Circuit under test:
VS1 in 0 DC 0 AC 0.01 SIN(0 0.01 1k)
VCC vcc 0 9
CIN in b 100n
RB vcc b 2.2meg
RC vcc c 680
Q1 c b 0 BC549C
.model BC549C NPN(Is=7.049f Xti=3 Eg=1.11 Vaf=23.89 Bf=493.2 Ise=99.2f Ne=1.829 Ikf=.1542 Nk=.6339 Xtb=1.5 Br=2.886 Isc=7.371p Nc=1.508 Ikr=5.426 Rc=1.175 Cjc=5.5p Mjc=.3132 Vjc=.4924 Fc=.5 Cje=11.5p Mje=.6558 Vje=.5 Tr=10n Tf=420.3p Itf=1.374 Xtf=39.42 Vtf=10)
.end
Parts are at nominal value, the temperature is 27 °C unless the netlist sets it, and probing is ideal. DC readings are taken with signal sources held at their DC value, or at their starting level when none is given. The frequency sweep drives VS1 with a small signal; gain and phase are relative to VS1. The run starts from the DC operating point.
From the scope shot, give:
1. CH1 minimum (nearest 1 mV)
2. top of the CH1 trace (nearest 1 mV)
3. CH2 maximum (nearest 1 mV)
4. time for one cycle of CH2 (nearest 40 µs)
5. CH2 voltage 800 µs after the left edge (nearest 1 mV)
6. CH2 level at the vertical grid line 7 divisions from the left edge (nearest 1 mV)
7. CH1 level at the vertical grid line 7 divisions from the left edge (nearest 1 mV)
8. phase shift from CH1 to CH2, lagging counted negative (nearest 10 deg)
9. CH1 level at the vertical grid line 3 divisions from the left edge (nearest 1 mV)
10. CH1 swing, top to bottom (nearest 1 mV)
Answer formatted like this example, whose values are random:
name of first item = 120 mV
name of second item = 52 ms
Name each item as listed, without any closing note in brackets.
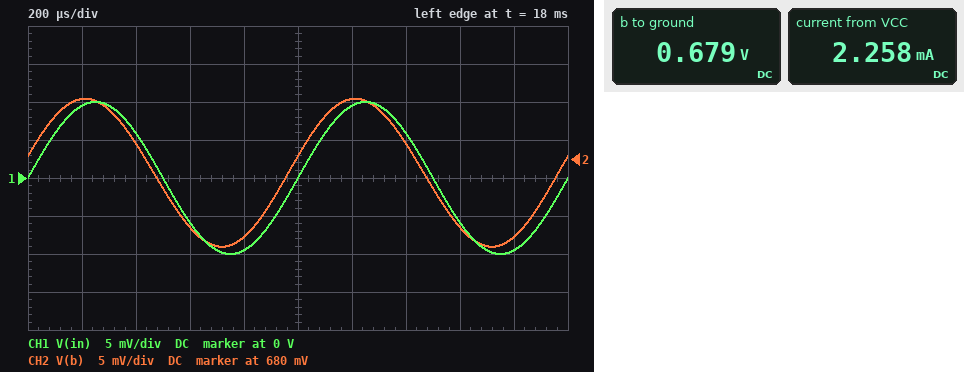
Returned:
CH1 minimum = -10 mV
top of the CH1 trace = 10 mV
CH2 maximum = 688 mV
time for one cycle of CH2 = 1.00 ms
CH2 voltage 800 µs after the left edge = 670 mV
CH2 level at the vertical grid line 7 divisions from the left edge = 682 mV
CH1 level at the vertical grid line 7 divisions from the left edge = 6 mV
phase shift from CH1 to CH2, lagging counted negative = 10 deg
CH1 level at the vertical grid line 3 divisions from the left edge = -6 mV
CH1 swing, top to bottom = 20 mV
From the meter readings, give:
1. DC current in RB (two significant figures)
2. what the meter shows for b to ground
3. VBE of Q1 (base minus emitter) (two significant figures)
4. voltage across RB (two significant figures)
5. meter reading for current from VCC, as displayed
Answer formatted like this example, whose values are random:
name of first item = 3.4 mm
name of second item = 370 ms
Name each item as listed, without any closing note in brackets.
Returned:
DC current in RB = 3.8 µA
what the meter shows for b to ground = 0.679 V
VBE of Q1 (base minus emitter) = 680 mV
voltage across RB = 8.3 V
meter reading for current from VCC, as displayed = 2.258 mA
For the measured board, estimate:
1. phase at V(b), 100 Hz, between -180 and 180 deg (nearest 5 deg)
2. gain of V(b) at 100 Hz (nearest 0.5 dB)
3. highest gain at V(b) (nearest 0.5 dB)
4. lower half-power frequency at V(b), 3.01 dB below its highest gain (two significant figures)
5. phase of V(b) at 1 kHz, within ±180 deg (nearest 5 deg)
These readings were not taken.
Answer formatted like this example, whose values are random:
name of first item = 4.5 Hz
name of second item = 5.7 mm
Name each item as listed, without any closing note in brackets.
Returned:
phase at V(b), 100 Hz, between -180 and 180 deg = 65 deg
gain of V(b) at 100 Hz = -8.0 dB
highest gain at V(b) = 0 dB
lower half-power frequency at V(b), 3.01 dB below its highest gain = 230 Hz
phase of V(b) at 1 kHz, within ±180 deg = 15 deg
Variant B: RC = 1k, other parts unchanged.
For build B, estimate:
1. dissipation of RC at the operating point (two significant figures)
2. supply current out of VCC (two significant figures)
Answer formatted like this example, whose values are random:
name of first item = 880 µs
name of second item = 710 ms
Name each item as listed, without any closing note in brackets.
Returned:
dissipation of RC at the operating point = 4.9 mW
supply current out of VCC = 2.2 mA
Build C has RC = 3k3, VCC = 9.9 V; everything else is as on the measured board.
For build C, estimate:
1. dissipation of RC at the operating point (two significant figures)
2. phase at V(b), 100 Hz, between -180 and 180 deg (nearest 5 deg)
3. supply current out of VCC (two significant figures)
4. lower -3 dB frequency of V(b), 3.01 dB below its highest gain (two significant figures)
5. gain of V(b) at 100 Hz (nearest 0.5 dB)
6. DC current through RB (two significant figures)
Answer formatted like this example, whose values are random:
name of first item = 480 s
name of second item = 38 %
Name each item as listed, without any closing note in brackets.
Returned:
dissipation of RC at the operating point = 15 mW
phase at V(b), 100 Hz, between -180 and 180 deg = 70 deg
supply current out of VCC = 2.1 mA
lower -3 dB frequency of V(b), 3.01 dB below its highest gain = 250 Hz
gain of V(b) at 100 Hz = -8.5 dB
DC current through RB = 4.2 µA
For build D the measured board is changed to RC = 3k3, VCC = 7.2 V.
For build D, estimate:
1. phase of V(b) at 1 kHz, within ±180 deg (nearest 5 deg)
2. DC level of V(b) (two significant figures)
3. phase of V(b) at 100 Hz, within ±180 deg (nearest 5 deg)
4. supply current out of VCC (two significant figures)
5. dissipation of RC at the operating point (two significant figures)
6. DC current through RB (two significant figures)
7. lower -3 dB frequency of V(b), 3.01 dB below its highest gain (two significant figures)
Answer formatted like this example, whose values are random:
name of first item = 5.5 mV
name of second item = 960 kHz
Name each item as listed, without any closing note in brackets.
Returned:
phase of V(b) at 1 kHz, within ±180 deg = 10 deg
DC level of V(b) = 670 mV
phase of V(b) at 100 Hz, within ±180 deg = 60 deg
supply current out of VCC = 1.5 mA
dissipation of RC at the operating point = 7.1 mW
DC current through RB = 3.0 µA
lower -3 dB frequency of V(b), 3.01 dB below its highest gain = 180 Hz
